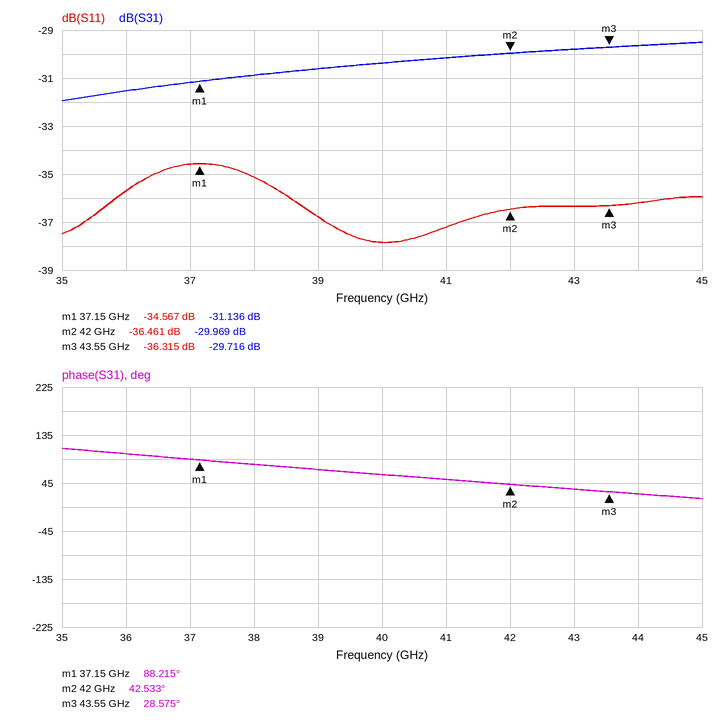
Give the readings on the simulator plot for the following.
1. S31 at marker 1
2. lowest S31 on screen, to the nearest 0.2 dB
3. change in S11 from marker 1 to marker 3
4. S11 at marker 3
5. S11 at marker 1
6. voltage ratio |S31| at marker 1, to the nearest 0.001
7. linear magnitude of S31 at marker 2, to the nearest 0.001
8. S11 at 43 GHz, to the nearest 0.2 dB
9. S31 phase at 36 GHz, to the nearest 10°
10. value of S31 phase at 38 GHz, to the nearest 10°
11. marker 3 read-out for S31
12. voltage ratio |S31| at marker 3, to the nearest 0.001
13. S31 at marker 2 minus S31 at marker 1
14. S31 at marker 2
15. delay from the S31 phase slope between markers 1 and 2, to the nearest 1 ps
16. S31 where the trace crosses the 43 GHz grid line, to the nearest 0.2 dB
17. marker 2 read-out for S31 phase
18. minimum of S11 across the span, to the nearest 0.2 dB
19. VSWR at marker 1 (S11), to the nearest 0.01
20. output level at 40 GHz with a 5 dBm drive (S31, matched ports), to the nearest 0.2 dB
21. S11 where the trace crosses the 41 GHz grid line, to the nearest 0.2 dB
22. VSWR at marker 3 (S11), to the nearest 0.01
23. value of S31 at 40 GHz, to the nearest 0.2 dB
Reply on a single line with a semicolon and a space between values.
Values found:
-31.136 dB; -32.0 dB; -1.748 dB; -36.315 dB; -34.567 dB; 0.028; 0.032; -36.4 dB; 100°; 80°; -29.716 dB; 0.033; 1.167 dB; -29.969 dB; 26 ps; -29.8 dB; 42.533°; -37.8 dB; 1.04; -25.4 dBm; -37.2 dB; 1.03; -30.4 dB
